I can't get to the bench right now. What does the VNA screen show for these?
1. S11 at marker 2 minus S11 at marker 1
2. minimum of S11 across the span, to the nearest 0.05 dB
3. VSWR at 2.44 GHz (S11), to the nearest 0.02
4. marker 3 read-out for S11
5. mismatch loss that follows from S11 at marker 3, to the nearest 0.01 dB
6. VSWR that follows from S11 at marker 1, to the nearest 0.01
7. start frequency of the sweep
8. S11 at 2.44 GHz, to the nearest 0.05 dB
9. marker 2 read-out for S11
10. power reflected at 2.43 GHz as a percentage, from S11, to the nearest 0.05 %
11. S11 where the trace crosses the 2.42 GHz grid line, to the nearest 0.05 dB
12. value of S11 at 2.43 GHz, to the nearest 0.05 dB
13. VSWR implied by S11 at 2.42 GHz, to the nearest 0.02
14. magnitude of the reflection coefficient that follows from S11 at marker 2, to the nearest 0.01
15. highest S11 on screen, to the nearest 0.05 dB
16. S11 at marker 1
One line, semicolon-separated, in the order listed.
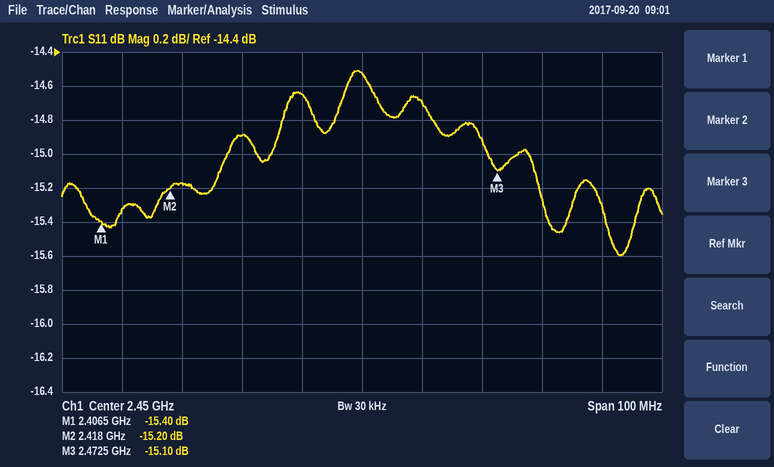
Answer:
0.20 dB; -15.60 dB; 1.46; -15.10 dB; 0.14 dB; 1.41; 2.4 GHz; -14.65 dB; -15.20 dB; 3.25 %; -15.15 dB; -14.90 dB; 1.42; 0.17; -14.50 dB; -15.40 dB
